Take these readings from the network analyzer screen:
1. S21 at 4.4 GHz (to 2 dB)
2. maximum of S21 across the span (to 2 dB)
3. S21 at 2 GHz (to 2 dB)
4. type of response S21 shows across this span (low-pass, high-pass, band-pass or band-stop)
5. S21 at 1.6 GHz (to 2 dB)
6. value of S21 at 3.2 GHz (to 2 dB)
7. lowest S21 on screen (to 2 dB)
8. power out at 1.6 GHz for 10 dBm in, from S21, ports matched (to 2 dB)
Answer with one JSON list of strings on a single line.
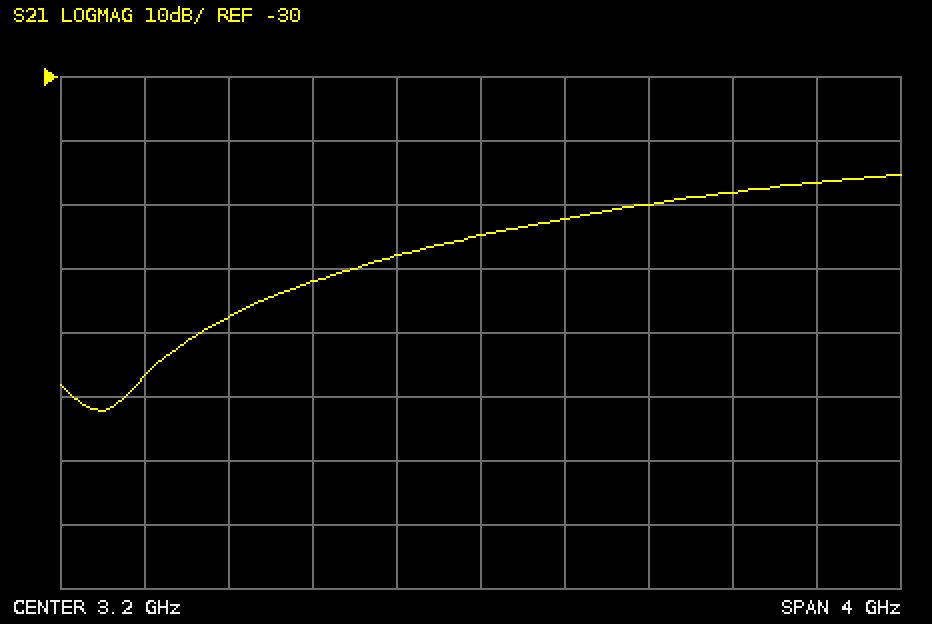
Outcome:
["-48 dB", "-46 dB", "-68 dB", "high-pass", "-76 dB", "-54 dB", "-82 dB", "-66 dBm"]
